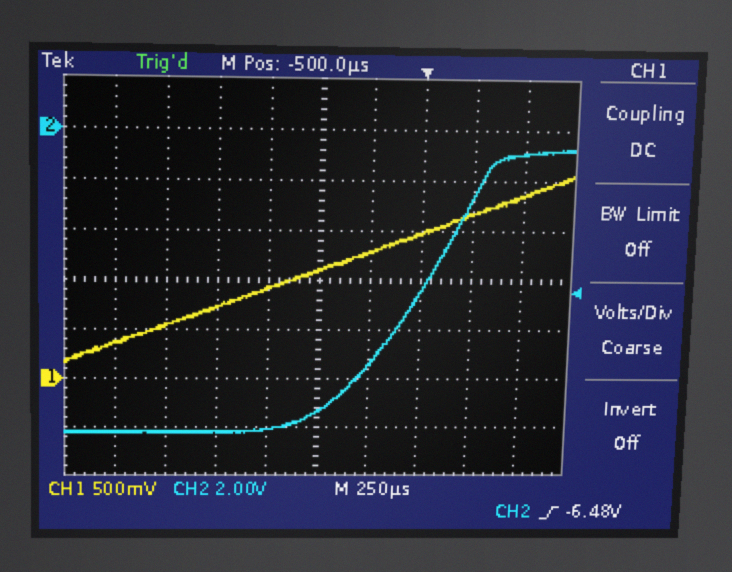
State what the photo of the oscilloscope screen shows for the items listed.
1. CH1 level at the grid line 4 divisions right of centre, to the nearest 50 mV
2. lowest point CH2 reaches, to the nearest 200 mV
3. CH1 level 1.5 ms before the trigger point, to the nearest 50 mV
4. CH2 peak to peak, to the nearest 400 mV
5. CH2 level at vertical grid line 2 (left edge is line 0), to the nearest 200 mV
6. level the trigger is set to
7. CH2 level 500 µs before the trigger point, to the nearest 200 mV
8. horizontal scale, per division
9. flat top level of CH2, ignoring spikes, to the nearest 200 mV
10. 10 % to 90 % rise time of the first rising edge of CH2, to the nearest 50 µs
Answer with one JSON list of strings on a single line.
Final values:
["1.85 V", "-12.2 V", "350 mV", "11.6 V", "-12.2 V", "-6.48 V", "-11.4 V", "250 µs", "-800 mV", "750 µs"]
